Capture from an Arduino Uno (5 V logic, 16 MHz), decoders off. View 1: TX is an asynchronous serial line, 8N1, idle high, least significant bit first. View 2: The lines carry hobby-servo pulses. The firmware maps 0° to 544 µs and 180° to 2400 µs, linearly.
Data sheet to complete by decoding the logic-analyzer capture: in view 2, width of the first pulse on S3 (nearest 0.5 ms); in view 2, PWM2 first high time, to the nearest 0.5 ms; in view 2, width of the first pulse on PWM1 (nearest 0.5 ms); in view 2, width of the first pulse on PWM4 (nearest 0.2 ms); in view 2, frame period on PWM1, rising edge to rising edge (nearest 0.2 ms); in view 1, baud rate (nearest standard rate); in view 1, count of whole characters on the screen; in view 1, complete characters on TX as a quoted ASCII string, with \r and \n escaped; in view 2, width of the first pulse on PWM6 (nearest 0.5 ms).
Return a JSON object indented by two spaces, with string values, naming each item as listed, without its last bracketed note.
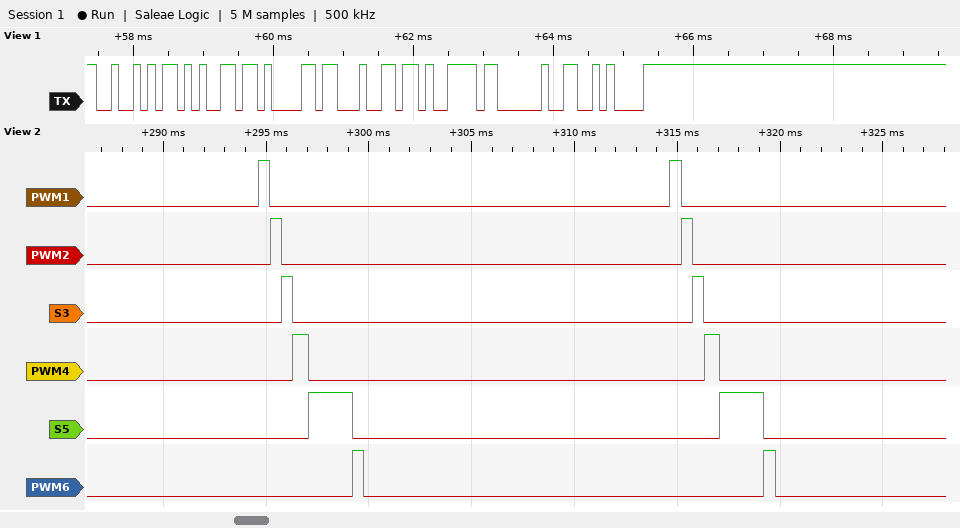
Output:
{
  "in view 2, width of the first pulse on S3": "0.5 ms",
  "in view 2, PWM2 first high time, to the nearest 0.5 ms": "0.5 ms",
  "in view 2, width of the first pulse on PWM1": "0.5 ms",
  "in view 2, width of the first pulse on PWM4": "0.8 ms",
  "in view 2, frame period on PWM1, rising edge to rising edge": "20.0 ms",
  "in view 1, baud rate": "9600 baud",
  "in view 1, count of whole characters on the screen": "7",
  "in view 1, complete characters on TX as a quoted ASCII string, with \\r and \\n escaped": "\"Ready \\n\"",
  "in view 2, width of the first pulse on PWM6": "0.5 ms"
}
